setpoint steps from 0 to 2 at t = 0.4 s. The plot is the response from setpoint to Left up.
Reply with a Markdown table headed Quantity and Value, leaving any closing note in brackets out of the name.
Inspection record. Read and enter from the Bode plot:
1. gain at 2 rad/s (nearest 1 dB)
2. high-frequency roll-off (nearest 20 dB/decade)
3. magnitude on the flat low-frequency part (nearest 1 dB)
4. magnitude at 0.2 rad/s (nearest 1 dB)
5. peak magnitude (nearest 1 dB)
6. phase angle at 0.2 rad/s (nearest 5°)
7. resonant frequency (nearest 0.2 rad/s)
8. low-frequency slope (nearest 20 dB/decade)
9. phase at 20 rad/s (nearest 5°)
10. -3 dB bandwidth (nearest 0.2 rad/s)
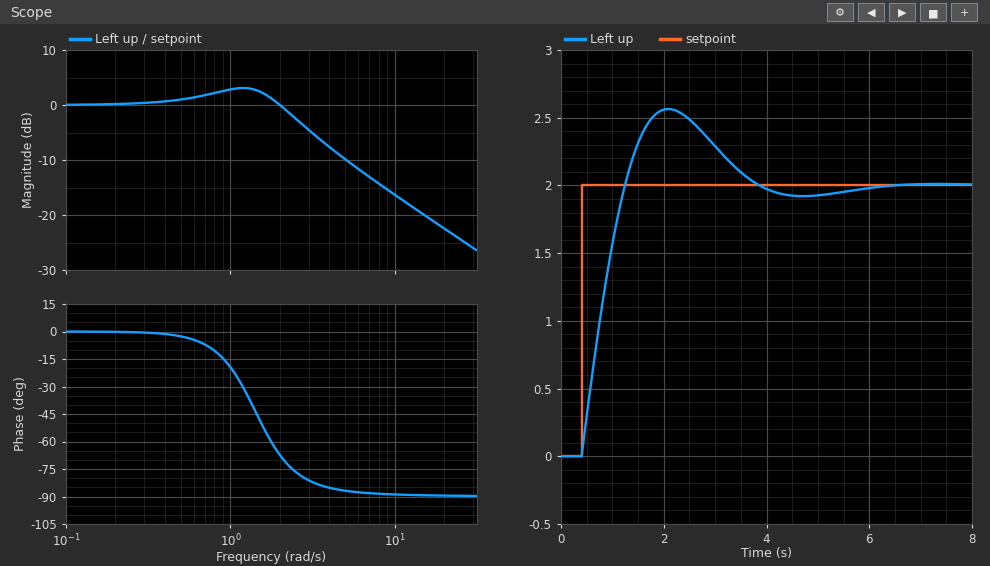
| Quantity | Value |
|---|---|
| gain at 2 rad/s | 0 dB |
| high-frequency roll-off | -20 dB/decade |
| magnitude on the flat low-frequency part | 0 dB |
| magnitude at 0.2 rad/s | 0 dB |
| peak magnitude | 3 dB |
| phase angle at 0.2 rad/s | 0° |
| resonant frequency | 1.2 rad/s |
| low-frequency slope | 0 dB/decade |
| phase at 20 rad/s | -90° |
| -3 dB bandwidth | 2.6 rad/s |
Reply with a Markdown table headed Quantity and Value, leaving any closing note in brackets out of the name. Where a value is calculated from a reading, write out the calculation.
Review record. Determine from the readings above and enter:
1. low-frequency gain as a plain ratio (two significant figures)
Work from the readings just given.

| Quantity | Value |
|---|---|
| low-frequency gain as a plain ratio | 10^(0 / 20) = 1.0 |
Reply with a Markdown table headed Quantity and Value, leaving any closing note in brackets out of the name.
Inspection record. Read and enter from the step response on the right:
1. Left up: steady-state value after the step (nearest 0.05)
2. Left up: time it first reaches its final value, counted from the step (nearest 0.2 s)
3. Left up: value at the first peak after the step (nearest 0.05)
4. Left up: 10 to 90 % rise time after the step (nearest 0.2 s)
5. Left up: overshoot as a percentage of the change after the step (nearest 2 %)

| Quantity | Value |
|---|---|
| Left up: steady-state value after the step | 2.00 |
| Left up: time it first reaches its final value, counted from the step | 0.8 s |
| Left up: value at the first peak after the step | 2.55 |
| Left up: 10 to 90 % rise time after the step | 0.6 s |
| Left up: overshoot as a percentage of the change after the step | 28 % |
